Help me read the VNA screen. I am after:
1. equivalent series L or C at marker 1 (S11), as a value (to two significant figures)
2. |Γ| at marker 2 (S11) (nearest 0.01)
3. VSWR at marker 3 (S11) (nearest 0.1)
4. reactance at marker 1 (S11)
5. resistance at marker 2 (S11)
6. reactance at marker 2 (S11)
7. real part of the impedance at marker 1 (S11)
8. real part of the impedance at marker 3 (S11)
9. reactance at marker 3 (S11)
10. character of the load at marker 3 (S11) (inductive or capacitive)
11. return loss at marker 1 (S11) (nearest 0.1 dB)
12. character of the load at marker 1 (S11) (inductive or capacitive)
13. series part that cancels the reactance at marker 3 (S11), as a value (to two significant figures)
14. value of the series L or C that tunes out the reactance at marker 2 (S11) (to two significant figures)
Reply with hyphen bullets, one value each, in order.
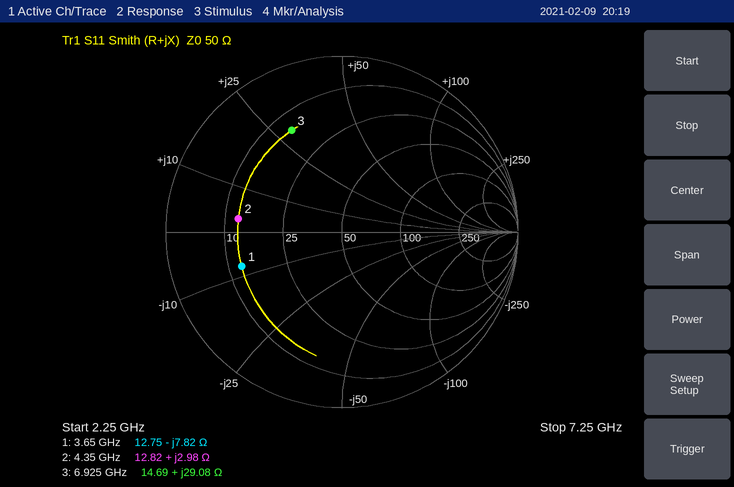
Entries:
- 5.6 pF
- 0.59
- 4.6
- -7.82 Ω
- 12.82 Ω
- +2.98 Ω
- 12.75 Ω
- 14.69 Ω
- +29.08 Ω
- inductive
- 4.4 dB
- capacitive
- 790 fF
- 12 pF
